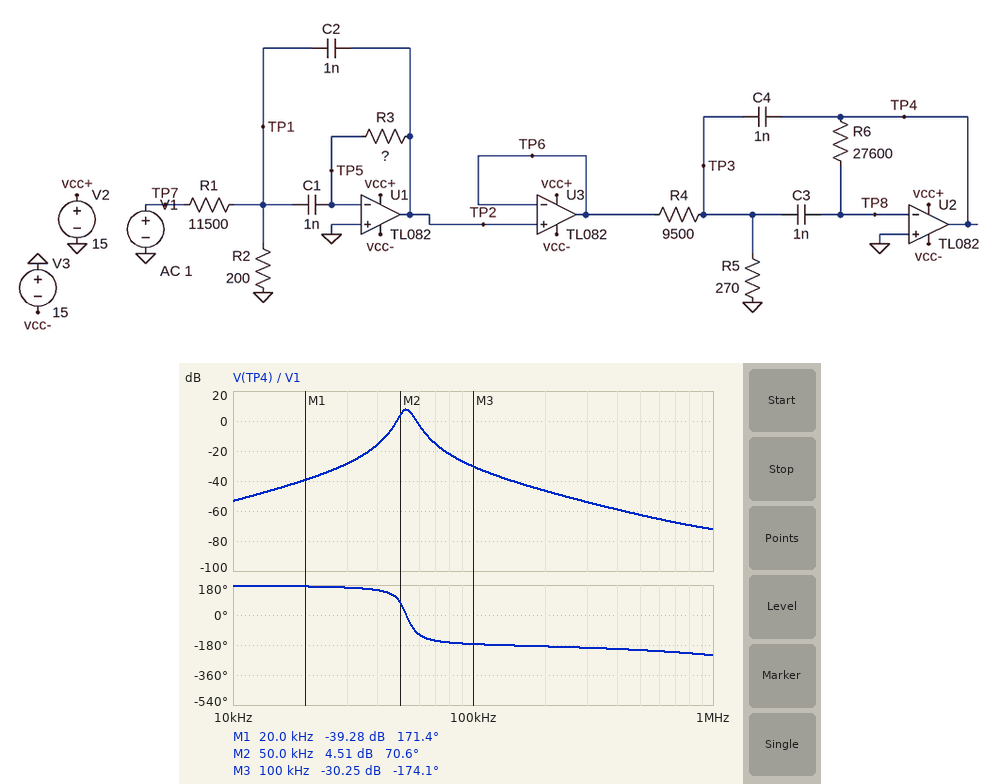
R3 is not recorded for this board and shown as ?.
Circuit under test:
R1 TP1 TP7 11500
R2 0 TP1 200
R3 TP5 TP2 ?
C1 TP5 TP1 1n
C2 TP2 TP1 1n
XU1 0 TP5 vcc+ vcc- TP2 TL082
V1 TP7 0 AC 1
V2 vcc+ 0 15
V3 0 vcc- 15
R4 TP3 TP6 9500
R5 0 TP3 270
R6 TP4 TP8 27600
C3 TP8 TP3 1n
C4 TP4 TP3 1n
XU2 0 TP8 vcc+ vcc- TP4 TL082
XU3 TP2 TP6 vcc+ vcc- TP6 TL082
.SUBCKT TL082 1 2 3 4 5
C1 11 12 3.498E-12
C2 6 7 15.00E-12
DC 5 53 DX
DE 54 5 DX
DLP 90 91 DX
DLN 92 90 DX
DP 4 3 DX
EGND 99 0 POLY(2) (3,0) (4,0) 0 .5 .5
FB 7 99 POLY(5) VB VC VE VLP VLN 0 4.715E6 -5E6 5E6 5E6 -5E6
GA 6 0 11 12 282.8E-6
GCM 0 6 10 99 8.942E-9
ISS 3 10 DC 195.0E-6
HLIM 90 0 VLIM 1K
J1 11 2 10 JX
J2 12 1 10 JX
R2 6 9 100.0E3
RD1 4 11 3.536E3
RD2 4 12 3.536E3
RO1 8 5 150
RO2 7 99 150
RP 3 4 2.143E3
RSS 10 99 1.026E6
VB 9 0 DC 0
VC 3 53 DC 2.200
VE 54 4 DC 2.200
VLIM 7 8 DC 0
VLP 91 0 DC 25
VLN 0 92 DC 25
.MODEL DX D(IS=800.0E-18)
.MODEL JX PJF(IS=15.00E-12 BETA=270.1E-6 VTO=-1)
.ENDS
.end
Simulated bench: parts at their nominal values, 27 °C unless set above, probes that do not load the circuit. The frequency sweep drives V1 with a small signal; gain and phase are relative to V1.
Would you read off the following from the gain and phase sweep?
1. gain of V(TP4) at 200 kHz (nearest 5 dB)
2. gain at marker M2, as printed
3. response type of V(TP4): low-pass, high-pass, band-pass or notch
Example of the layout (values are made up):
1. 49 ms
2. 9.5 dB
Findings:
1. -45 dB
2. 4.51 dB
3. band-pass
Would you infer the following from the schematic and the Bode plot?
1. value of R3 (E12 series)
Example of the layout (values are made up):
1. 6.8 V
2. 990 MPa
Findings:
1. 39 kΩ
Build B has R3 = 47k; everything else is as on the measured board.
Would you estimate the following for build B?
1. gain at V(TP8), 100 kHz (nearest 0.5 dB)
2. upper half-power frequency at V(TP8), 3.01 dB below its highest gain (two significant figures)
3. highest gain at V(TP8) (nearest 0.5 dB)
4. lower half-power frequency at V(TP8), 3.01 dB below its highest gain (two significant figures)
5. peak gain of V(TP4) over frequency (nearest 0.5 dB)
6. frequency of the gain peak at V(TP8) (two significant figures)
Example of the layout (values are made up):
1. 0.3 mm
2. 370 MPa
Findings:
1. -61.5 dB
2. 55 kHz
3. -32.0 dB
4. 46 kHz
5. 5.0 dB
6. 48 kHz
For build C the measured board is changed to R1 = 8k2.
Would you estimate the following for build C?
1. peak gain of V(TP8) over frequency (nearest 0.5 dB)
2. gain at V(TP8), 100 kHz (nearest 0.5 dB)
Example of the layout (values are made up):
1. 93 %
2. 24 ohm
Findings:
1. -25.5 dB
2. -58.0 dB
